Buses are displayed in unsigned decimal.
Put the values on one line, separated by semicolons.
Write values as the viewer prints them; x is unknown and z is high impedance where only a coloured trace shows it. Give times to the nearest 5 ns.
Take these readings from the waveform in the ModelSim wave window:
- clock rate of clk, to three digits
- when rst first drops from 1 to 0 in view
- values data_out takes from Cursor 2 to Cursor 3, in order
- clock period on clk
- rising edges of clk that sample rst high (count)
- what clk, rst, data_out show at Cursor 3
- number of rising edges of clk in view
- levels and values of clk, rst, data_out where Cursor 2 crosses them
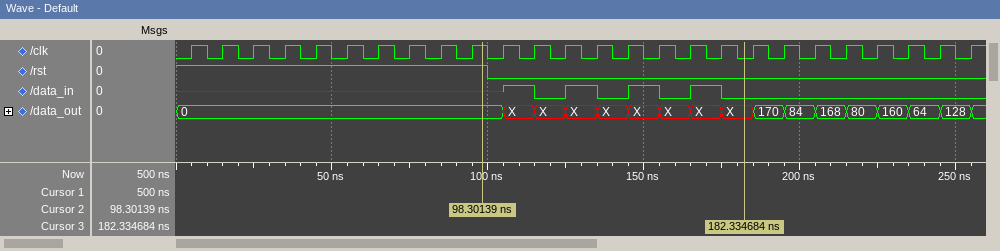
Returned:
100 MHz; 100 ns; 0, X, X, X, X, X, X, X, X; 10 ns; 10; clk=0, rst=0, data_out=X; 26; clk=1, rst=1, data_out=0
